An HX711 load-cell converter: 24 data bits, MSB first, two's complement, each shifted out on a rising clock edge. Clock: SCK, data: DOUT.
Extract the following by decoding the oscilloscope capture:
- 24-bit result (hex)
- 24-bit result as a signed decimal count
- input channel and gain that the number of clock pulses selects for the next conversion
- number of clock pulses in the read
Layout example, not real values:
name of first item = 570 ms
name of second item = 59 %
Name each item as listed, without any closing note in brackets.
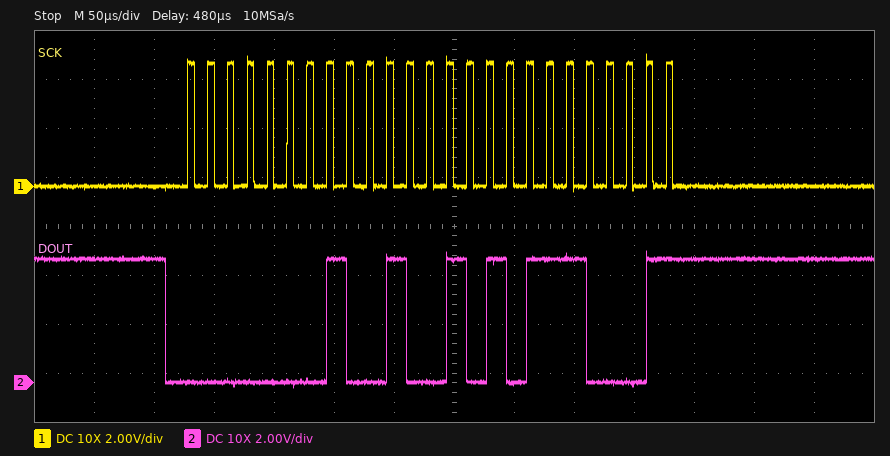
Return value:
24-bit result = 0x012571
24-bit result as a signed decimal count = 75121
input channel and gain that the number of clock pulses selects for the next conversion = channel A, gain 128
number of clock pulses in the read = 25
